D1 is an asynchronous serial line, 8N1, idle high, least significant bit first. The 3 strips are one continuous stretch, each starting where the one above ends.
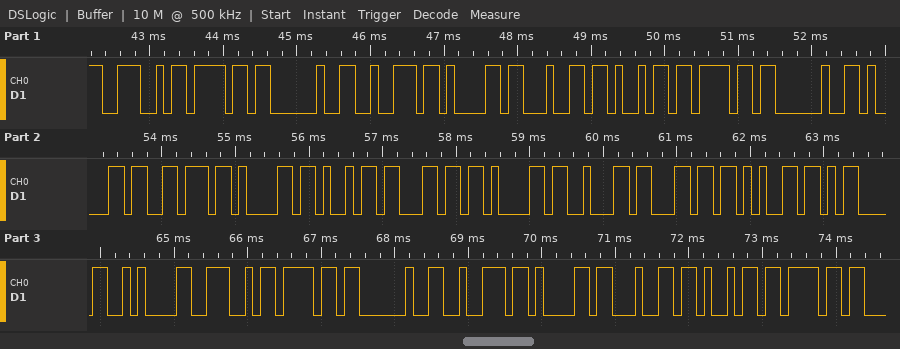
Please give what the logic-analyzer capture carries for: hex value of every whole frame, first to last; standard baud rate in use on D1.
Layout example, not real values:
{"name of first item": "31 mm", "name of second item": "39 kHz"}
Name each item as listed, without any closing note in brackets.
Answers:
{"hex value of every whole frame, first to last": "4E 6F 20 72 61 64 69 6F 20 61 76 61 69 6C 61 62 6C 65 0D 0A 4E 6F 20 72 61 64 69 6F", "standard baud rate in use on D1": "9600 baud"}
